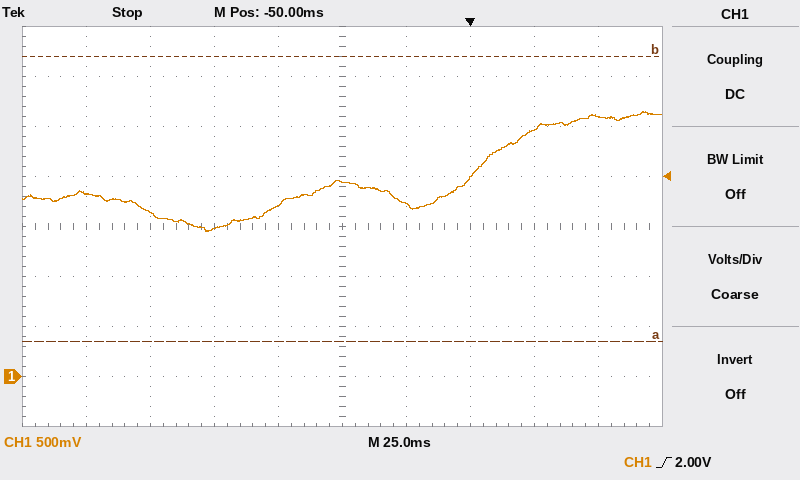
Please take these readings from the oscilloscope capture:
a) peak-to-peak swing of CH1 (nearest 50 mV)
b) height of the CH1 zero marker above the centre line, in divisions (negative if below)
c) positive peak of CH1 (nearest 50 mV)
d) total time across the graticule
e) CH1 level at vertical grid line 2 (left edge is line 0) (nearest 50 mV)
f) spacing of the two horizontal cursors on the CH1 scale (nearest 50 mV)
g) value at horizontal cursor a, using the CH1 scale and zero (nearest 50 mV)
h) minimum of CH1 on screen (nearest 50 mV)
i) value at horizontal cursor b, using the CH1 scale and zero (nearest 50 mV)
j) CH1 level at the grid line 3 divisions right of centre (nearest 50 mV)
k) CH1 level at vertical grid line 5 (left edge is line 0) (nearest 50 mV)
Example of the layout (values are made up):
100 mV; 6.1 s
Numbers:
1.20 V; -3.0 div; 2.65 V; 250 ms; 1.65 V; 2.85 V; 350 mV; 1.45 V; 3.20 V; 2.45 V; 1.95 V
